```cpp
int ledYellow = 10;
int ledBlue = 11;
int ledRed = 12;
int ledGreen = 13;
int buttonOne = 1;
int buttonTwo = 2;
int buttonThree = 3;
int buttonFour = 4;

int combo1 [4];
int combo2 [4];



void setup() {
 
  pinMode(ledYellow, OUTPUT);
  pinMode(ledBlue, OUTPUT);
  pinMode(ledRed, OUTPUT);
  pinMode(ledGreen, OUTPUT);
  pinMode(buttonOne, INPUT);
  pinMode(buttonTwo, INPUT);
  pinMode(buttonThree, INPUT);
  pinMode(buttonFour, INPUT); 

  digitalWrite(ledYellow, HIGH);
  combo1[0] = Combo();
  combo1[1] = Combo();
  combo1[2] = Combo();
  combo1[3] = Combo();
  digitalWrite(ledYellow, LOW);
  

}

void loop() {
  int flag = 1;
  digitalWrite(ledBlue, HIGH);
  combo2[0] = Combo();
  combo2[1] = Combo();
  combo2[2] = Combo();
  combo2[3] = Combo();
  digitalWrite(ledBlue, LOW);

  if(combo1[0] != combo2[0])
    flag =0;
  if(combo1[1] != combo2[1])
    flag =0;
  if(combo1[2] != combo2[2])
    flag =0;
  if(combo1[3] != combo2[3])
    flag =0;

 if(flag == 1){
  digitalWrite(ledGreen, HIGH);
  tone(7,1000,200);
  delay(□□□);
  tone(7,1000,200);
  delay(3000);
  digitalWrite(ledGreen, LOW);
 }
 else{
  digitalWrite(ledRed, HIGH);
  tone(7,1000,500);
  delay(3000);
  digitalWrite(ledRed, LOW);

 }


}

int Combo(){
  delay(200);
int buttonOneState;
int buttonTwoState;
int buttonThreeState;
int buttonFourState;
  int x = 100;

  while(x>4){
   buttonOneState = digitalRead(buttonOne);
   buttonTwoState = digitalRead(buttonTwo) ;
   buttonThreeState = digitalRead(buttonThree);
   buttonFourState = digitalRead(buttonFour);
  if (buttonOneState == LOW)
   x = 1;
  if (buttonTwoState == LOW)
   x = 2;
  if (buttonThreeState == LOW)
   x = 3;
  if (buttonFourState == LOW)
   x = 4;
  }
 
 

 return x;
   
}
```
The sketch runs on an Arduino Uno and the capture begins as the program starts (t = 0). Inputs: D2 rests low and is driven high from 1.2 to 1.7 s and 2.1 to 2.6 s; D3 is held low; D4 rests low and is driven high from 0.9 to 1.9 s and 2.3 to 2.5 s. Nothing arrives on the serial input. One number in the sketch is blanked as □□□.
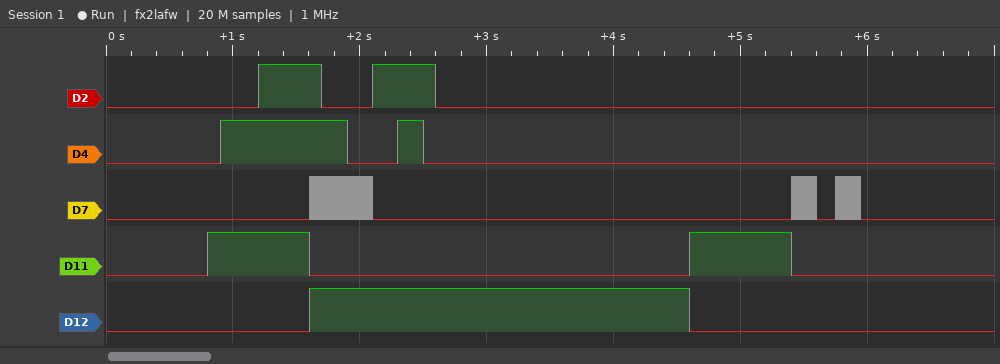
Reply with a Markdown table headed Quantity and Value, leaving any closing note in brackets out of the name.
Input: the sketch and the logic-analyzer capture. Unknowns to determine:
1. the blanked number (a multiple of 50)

| Quantity | Value |
|---|---|
| the blanked number | 350 |
